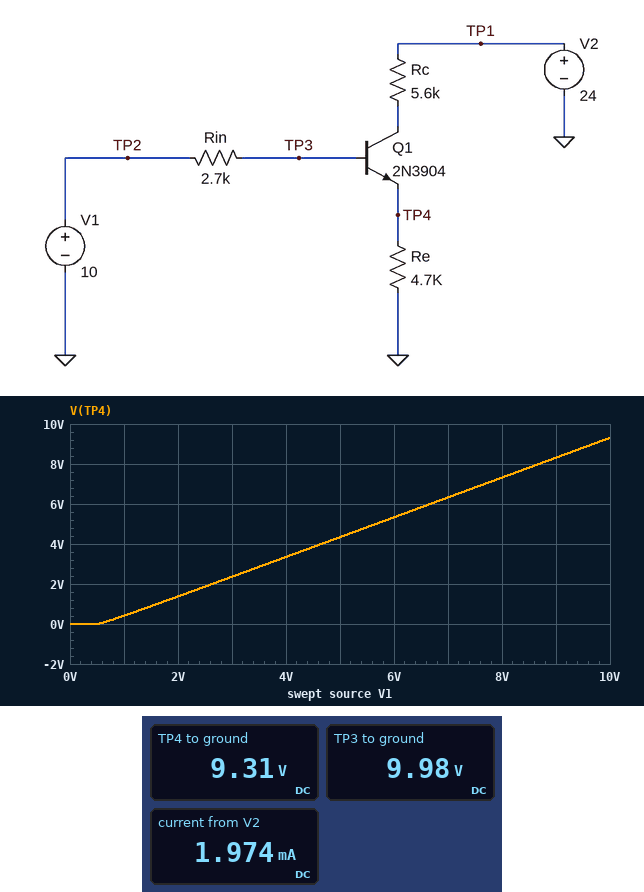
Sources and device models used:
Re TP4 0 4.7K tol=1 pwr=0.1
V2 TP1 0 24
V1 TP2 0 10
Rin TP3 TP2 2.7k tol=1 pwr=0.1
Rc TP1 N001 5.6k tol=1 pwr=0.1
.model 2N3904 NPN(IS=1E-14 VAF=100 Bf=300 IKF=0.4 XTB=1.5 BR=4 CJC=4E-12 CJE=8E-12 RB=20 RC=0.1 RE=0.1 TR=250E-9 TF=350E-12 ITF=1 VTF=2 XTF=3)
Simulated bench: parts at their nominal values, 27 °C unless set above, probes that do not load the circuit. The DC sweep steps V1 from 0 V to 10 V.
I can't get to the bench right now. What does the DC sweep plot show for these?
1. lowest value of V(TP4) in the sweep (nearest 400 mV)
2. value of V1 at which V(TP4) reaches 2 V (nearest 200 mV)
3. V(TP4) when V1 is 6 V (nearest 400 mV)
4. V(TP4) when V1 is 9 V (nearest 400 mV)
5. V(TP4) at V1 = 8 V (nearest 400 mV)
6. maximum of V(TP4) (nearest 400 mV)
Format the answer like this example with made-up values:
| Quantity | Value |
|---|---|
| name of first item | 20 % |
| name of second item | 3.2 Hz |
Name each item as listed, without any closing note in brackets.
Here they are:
| Quantity | Value |
|---|---|
| lowest value of V(TP4) in the sweep | 0 V |
| value of V1 at which V(TP4) reaches 2 V | 2.6 V |
| V(TP4) when V1 is 6 V | 5.2 V |
| V(TP4) when V1 is 9 V | 8.4 V |
| V(TP4) at V1 = 8 V | 7.2 V |
| maximum of V(TP4) | 9.2 V |
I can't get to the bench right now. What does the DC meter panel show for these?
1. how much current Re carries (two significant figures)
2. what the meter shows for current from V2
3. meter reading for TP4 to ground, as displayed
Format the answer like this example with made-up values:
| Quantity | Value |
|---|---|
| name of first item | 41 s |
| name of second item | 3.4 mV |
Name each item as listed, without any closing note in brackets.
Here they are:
| Quantity | Value |
|---|---|
| how much current Re carries | 2.0 mA |
| what the meter shows for current from V2 | 1.974 mA |
| meter reading for TP4 to ground, as displayed | 9.31 V |
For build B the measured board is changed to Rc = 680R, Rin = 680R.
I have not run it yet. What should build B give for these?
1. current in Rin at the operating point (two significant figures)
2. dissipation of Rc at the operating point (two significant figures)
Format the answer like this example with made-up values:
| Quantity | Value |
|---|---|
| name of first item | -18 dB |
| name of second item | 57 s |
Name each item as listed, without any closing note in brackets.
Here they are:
| Quantity | Value |
|---|---|
| current in Rin at the operating point | 5.9 µA |
| dissipation of Rc at the operating point | 2.7 mW |
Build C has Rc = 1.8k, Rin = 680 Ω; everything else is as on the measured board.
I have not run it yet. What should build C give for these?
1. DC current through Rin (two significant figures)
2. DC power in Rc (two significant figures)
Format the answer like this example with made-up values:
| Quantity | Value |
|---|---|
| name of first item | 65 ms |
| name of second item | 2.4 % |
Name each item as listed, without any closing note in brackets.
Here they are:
| Quantity | Value |
|---|---|
| DC current through Rin | 6.0 µA |
| DC power in Rc | 7.0 mW |
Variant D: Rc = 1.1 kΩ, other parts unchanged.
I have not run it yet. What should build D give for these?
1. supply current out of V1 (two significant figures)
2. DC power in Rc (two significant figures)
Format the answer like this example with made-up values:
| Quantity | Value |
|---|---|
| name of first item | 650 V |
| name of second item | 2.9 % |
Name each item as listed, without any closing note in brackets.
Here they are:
| Quantity | Value |
|---|---|
| supply current out of V1 | 5.9 µA |
| DC power in Rc | 4.3 mW |
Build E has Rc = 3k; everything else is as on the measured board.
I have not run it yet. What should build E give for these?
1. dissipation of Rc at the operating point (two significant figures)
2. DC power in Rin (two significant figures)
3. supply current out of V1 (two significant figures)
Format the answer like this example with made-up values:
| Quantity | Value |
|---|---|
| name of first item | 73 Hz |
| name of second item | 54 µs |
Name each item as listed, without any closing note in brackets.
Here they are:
| Quantity | Value |
|---|---|
| dissipation of Rc at the operating point | 12 mW |
| DC power in Rin | 100 nW |
| supply current out of V1 | 6.1 µA |
